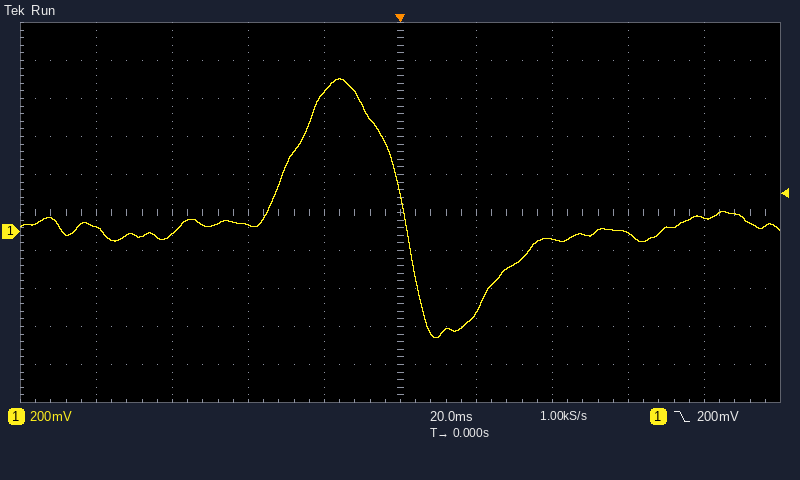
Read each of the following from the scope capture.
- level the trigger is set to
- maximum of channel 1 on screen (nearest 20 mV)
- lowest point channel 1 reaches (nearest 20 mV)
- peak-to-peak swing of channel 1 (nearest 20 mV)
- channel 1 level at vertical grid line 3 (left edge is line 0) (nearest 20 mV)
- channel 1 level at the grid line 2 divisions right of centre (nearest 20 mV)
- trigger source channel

200 mV
800 mV
-560 mV
1.36 V
40 mV
-40 mV
channel 1
